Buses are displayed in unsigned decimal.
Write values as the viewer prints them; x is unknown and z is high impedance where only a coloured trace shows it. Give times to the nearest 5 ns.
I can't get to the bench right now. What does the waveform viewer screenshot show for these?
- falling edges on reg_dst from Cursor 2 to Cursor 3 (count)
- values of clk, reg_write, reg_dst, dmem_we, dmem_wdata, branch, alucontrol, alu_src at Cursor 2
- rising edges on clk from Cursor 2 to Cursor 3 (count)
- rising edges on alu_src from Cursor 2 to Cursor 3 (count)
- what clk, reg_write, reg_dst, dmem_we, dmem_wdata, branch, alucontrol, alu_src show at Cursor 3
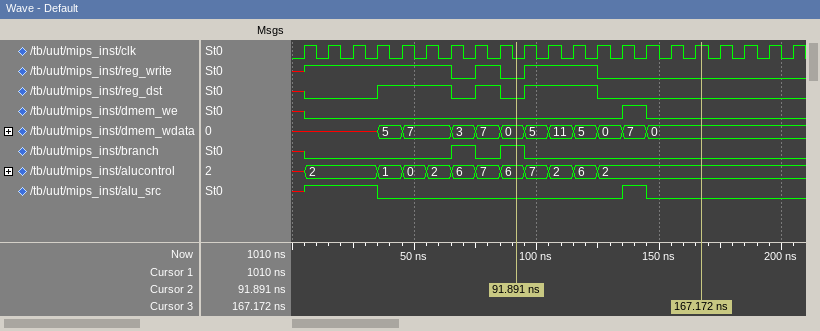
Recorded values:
1
clk=0, reg_write=0, reg_dst=0, dmem_we=0, dmem_wdata=0, branch=1, alucontrol=6, alu_src=0
8
1
clk=1, reg_write=0, reg_dst=0, dmem_we=0, dmem_wdata=0, branch=0, alucontrol=2, alu_src=0
